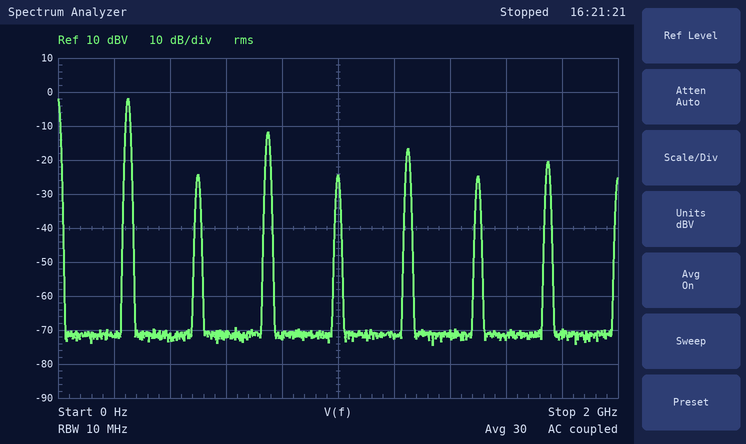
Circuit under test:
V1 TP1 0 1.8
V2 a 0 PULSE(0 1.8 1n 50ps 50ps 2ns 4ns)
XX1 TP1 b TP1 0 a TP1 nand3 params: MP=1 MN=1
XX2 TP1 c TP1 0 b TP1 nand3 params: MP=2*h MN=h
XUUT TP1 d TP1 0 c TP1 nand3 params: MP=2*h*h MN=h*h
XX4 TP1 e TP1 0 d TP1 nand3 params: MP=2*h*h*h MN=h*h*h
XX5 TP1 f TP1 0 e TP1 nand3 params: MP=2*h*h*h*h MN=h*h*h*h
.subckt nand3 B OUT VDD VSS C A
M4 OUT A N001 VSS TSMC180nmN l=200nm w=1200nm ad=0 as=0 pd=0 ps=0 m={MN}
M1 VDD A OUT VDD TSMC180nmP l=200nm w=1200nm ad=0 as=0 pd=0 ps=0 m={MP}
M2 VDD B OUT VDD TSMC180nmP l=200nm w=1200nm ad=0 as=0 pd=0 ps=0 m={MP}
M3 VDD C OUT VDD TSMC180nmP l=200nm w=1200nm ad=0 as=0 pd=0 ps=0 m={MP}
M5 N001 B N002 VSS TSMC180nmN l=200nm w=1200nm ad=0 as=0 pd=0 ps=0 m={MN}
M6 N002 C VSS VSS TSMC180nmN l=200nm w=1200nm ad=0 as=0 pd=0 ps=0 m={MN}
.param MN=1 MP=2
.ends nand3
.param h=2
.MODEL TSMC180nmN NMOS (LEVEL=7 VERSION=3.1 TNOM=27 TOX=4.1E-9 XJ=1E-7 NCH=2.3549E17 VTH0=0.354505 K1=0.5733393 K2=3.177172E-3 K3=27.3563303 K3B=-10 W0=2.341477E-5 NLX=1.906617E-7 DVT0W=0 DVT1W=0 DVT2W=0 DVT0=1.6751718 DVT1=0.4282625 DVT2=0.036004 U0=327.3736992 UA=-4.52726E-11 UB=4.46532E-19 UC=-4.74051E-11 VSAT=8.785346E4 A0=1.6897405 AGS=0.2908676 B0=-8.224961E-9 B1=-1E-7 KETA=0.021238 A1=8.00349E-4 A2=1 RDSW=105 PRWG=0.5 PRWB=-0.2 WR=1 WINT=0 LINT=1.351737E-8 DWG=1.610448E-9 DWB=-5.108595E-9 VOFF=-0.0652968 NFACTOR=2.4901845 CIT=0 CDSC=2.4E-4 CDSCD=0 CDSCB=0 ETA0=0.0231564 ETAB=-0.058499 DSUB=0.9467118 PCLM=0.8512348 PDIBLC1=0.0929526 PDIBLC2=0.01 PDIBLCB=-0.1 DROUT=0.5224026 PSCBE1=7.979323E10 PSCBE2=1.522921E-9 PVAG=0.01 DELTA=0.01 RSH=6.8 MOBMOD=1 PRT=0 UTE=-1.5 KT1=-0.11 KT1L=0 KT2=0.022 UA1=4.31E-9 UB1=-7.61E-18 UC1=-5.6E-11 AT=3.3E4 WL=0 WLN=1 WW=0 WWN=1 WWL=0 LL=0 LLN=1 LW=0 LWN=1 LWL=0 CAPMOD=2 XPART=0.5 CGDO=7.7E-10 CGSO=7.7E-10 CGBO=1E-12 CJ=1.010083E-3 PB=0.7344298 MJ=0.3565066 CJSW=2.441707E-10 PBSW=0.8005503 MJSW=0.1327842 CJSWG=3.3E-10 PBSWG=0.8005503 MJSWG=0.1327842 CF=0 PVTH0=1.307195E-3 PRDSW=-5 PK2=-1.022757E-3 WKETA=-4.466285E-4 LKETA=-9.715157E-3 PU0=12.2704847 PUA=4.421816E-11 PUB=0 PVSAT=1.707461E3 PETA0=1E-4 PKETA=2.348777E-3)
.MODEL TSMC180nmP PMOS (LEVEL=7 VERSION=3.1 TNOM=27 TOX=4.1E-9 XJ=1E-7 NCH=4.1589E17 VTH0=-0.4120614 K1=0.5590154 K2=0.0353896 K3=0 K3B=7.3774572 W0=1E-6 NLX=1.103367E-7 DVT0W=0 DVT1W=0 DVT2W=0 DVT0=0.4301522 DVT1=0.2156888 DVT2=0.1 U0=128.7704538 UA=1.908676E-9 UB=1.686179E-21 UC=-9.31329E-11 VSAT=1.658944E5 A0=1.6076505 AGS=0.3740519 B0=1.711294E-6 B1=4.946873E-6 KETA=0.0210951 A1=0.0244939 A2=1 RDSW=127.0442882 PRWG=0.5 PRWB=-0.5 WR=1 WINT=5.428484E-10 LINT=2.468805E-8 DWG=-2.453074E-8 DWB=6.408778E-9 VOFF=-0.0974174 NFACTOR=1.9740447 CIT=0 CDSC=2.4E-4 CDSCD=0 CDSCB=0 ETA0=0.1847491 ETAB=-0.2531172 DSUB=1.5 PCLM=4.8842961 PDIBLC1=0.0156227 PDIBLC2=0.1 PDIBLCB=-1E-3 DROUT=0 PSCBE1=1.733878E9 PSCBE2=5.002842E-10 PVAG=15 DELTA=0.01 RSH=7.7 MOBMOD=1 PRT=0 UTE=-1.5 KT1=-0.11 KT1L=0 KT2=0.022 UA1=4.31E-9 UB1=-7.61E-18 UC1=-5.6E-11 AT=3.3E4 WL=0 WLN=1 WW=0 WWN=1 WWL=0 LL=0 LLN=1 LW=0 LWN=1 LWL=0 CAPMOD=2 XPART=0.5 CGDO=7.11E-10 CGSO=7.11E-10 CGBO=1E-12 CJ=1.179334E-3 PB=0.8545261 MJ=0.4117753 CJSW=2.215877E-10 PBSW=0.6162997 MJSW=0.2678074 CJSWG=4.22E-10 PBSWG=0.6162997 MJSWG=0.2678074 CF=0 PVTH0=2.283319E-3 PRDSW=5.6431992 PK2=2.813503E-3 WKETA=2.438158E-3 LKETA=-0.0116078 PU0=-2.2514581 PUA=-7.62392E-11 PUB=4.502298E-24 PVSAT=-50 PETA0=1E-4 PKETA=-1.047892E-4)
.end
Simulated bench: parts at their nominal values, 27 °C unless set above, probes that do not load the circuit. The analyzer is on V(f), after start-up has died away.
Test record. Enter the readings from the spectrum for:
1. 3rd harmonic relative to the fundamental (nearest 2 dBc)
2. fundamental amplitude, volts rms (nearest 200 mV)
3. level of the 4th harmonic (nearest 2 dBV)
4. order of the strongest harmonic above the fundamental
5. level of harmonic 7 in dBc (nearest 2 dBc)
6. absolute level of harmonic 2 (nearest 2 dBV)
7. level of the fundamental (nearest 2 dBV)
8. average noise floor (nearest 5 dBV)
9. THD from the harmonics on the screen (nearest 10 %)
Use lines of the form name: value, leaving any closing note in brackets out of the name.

3rd harmonic relative to the fundamental: -10 dBc
fundamental amplitude, volts rms: 800 mV
level of the 4th harmonic: -24 dBV
order of the strongest harmonic above the fundamental: 3
level of harmonic 7 in dBc: -18 dBc
absolute level of harmonic 2: -24 dBV
level of the fundamental: -2 dBV
average noise floor: -70 dBV
THD from the harmonics on the screen: 40 %
